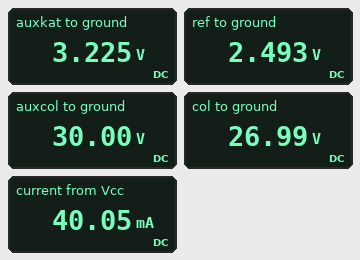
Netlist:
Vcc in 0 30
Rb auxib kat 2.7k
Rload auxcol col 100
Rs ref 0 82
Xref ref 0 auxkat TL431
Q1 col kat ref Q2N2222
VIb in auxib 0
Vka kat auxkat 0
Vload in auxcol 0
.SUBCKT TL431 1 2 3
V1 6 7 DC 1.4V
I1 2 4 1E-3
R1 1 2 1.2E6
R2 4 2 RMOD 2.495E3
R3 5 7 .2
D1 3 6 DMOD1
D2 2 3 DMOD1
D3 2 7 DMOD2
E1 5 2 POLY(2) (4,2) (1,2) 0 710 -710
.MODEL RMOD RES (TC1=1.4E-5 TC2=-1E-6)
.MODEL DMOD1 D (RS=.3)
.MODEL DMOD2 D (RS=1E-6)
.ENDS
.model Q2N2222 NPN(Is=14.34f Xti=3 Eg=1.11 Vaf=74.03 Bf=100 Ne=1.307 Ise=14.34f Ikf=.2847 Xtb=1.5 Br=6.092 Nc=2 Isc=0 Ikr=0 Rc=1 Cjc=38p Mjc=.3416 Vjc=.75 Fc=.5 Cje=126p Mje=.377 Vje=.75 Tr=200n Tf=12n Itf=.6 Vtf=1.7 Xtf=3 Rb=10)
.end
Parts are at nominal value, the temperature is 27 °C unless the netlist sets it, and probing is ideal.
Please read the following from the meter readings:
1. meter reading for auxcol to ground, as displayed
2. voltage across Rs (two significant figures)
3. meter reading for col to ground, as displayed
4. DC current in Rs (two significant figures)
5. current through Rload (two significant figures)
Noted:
30.00 V
2.5 V
26.99 V
30 mA
30 mA
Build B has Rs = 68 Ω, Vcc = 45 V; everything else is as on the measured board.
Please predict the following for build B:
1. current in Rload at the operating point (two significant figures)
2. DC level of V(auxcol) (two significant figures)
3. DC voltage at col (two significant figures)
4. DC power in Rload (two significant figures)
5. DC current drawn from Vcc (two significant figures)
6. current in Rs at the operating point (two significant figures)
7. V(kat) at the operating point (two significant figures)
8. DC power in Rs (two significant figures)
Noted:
36 mA
45 V
41 V
130 mW
52 mA
37 mA
3.2 V
91 mW
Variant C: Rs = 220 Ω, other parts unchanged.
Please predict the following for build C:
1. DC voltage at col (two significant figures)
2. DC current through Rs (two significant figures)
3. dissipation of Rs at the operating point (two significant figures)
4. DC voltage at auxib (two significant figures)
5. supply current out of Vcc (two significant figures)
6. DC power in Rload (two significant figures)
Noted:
29 V
11 mA
28 mW
30 V
21 mA
13 mW
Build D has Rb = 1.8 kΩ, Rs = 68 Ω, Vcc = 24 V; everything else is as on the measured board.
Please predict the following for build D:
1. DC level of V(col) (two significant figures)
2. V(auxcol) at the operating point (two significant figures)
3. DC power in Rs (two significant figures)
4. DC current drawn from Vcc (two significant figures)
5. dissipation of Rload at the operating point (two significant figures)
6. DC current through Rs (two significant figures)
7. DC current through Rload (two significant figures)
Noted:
20 V
24 V
91 mW
48 mA
130 mW
37 mA
36 mA
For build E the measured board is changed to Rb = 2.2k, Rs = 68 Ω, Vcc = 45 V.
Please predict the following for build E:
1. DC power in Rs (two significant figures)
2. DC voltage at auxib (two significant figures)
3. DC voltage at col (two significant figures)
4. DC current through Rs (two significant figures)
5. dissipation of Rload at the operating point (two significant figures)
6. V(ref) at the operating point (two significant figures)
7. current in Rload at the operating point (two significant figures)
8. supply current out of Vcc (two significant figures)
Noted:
91 mW
45 V
41 V
37 mA
130 mW
2.5 V
36 mA
55 mA
